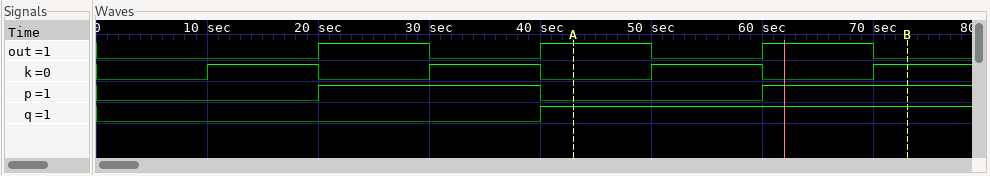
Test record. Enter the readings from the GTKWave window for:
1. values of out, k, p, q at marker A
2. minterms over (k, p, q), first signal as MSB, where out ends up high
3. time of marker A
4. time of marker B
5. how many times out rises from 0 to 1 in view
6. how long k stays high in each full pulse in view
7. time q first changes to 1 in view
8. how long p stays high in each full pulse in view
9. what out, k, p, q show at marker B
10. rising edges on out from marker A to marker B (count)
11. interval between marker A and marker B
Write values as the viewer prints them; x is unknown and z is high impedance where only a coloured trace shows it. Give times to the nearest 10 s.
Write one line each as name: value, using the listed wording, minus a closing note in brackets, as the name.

values of out, k, p, q at marker A: out=1, k=0, p=0, q=1
minterms over (k, p, q), first signal as MSB, where out ends up high: 1, 2, 3
time of marker A: 40 s
time of marker B: 70 s
how many times out rises from 0 to 1 in view: 3
how long k stays high in each full pulse in view: 10 s, 10 s, 10 s
time q first changes to 1 in view: 40 s
how long p stays high in each full pulse in view: 20 s
what out, k, p, q show at marker B: out=0, k=1, p=1, q=1
rising edges on out from marker A to marker B: 1
interval between marker A and marker B: 30 s
